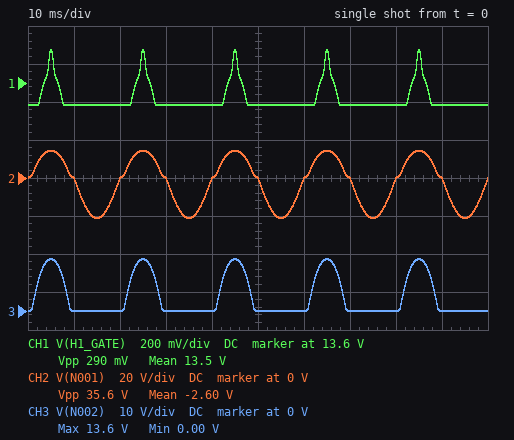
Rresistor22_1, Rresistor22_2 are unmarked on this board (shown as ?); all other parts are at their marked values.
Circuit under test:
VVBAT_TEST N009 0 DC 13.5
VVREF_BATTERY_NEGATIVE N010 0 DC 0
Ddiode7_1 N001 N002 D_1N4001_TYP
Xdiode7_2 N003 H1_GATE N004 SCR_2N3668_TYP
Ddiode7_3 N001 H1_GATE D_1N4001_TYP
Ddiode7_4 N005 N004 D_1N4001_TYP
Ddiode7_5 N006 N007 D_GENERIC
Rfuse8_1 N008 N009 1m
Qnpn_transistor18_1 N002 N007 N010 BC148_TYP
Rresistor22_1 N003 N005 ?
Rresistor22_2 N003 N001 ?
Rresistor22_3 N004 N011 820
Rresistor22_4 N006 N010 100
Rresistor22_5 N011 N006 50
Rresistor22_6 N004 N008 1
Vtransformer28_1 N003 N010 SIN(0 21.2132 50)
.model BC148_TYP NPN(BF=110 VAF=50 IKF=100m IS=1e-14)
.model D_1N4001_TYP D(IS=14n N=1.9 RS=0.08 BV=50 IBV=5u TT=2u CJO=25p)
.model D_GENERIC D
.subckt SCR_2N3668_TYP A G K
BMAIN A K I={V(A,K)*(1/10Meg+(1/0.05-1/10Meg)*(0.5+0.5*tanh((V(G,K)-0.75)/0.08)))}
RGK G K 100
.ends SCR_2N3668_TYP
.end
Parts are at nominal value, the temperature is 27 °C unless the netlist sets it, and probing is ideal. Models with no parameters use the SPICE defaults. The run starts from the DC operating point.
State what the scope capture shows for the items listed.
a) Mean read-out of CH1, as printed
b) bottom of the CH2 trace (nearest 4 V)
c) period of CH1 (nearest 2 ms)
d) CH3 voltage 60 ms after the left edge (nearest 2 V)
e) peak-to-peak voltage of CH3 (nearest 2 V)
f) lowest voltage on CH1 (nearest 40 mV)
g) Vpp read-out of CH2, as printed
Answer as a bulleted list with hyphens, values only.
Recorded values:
- 13.5 V
- -20 V
- 20 ms
- 0 V
- 14 V
- 13.48 V
- 35.6 V
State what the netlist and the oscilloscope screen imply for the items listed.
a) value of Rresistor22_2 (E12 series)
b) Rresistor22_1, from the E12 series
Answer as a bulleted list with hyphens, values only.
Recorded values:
- 180 Ω
- 39 Ω
